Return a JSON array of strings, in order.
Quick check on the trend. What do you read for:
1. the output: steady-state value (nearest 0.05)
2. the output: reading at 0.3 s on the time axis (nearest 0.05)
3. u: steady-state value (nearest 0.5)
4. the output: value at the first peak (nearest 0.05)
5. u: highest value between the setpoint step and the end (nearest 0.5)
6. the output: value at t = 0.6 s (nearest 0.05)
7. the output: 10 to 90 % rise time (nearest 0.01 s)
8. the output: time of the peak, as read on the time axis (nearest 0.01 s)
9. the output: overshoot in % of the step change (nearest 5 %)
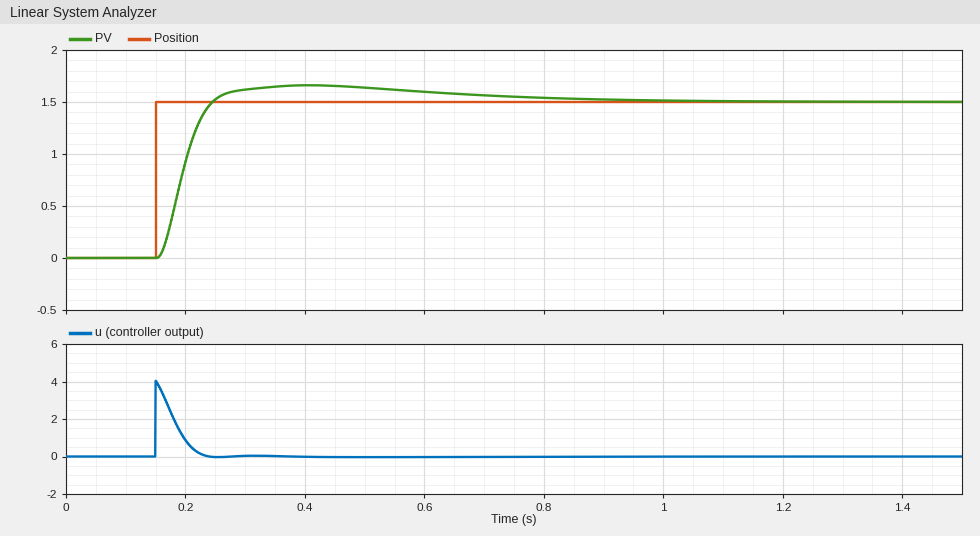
["1.50", "1.60", "0.0", "1.65", "4.0", "1.60", "0.06 s", "0.41 s", "10 %"]
